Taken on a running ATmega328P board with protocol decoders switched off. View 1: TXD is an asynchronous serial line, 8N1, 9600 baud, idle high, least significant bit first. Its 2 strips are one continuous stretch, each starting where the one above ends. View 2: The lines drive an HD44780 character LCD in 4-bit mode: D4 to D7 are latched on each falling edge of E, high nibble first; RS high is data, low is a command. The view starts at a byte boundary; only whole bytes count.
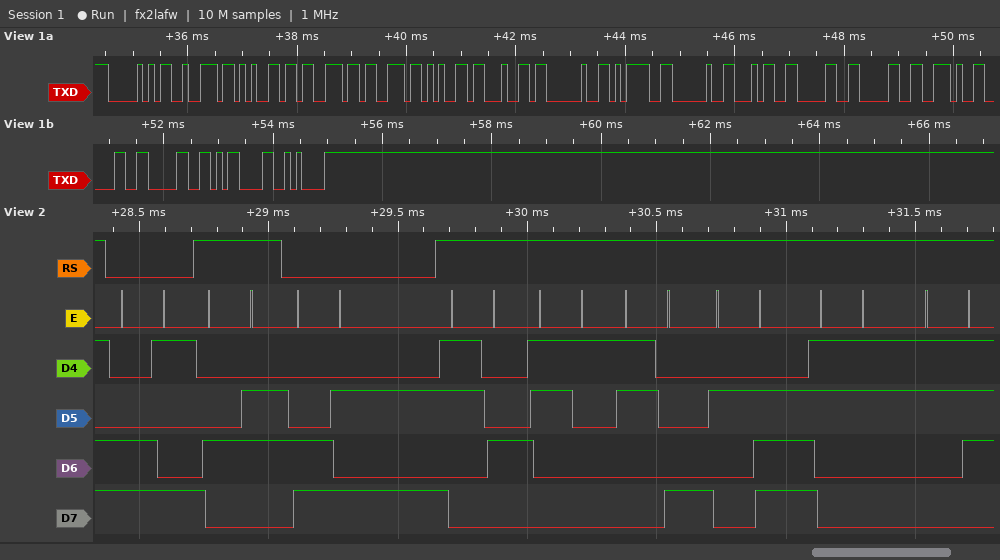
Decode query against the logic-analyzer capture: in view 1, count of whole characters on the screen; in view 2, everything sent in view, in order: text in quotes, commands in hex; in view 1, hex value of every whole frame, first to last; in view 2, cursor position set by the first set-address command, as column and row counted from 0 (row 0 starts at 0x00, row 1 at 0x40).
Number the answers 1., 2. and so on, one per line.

1. 18
2. 0xC9 "F" 0xCA "418.37"
3. 50 72 65 73 73 65 64 20 3D 20 34 30 30 2E 30 30 0D 0A
4. column 9, row 1
